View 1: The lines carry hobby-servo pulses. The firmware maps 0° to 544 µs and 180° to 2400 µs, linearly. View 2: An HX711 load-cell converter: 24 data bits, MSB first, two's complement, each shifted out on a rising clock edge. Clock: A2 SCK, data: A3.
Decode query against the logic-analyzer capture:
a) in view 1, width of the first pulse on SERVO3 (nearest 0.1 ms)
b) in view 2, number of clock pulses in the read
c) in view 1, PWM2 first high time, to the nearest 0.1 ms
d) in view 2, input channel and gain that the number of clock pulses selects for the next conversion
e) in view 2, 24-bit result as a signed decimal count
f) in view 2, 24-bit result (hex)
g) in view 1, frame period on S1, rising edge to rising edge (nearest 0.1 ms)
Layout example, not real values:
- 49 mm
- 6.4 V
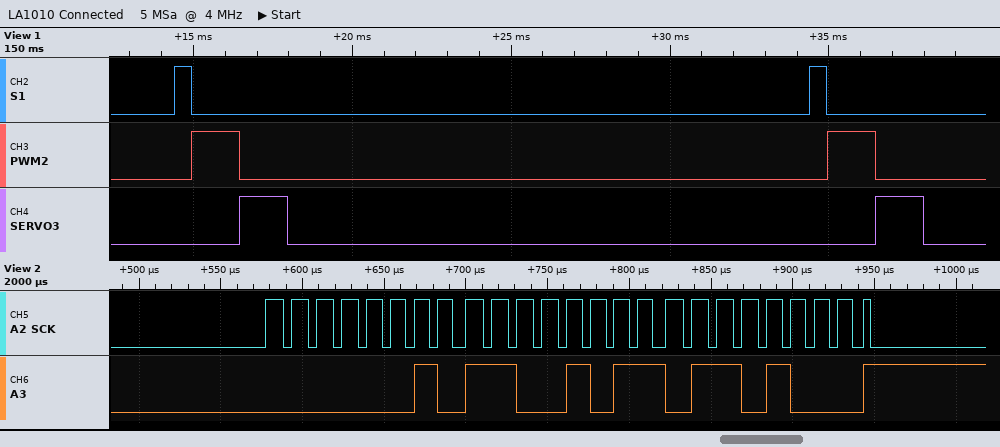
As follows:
- 1.5 ms
- 25
- 1.5 ms
- channel A, gain 128
- 183144
- 0x02CB68
- 20.0 ms
